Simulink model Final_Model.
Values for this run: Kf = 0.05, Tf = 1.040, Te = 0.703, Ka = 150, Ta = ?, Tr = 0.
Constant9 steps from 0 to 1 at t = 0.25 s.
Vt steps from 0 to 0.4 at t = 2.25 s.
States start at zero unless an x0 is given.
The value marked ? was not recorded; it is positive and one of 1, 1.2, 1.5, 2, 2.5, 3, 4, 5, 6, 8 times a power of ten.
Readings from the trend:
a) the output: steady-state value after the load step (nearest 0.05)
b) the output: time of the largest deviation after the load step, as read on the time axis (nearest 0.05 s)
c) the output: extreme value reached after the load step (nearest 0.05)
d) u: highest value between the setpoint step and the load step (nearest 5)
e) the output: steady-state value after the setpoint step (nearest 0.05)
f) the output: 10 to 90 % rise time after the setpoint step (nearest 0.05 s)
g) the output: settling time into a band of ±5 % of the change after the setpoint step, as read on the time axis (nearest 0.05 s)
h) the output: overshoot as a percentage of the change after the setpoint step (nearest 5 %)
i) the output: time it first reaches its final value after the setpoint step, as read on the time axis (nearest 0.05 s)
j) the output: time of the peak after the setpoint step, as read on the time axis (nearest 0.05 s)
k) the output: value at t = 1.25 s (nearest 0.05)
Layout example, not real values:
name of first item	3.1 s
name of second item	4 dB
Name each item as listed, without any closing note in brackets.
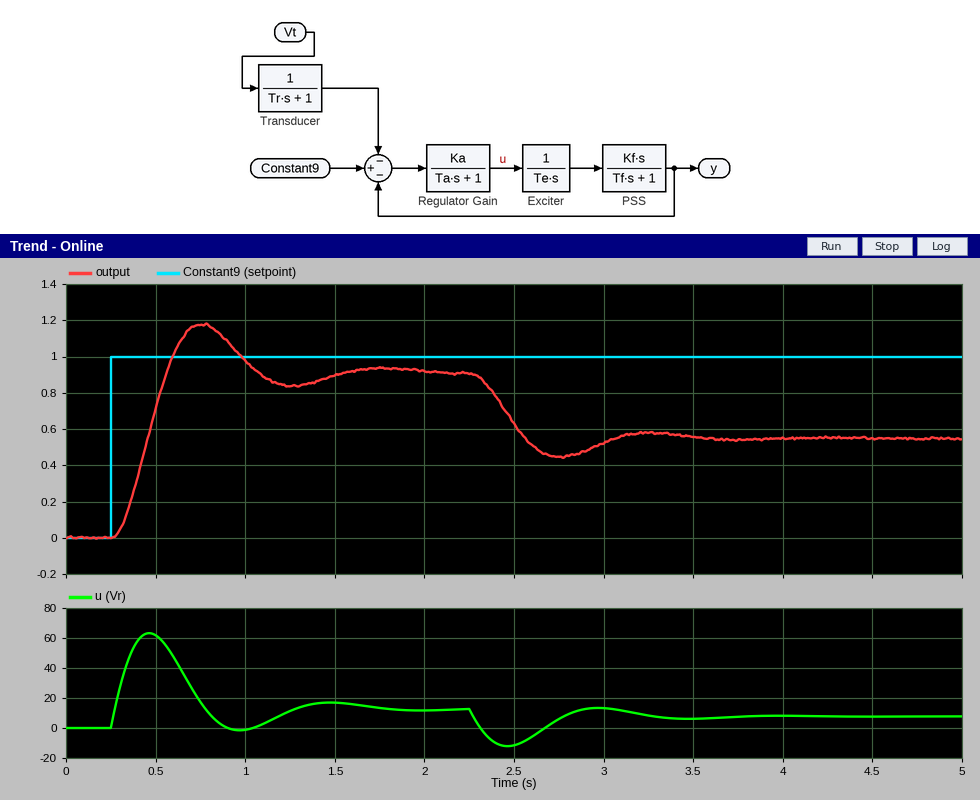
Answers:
the output: steady-state value after the load step	0.55
the output: time of the largest deviation after the load step, as read on the time axis	2.75 s
the output: extreme value reached after the load step	0.45
u: highest value between the setpoint step and the load step	65
the output: steady-state value after the setpoint step	0.90
the output: 10 to 90 % rise time after the setpoint step	0.20 s
the output: settling time into a band of ±5 % of the change after the setpoint step, as read on the time axis	1.40 s
the output: overshoot as a percentage of the change after the setpoint step	30 %
the output: time it first reaches its final value after the setpoint step, as read on the time axis	0.55 s
the output: time of the peak after the setpoint step, as read on the time axis	0.75 s
the output: value at t = 1.25 s	0.85
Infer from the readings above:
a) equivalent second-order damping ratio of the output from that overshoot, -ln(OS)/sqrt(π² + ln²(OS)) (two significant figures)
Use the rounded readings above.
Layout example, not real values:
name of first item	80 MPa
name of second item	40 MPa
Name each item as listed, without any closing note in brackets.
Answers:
equivalent second-order damping ratio of the output from that overshoot, -ln(OS)/sqrt(π² + ln²(OS))	0.36
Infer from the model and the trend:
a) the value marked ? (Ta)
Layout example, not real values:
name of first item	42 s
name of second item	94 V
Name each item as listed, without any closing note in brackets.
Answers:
the value marked ?	0.25
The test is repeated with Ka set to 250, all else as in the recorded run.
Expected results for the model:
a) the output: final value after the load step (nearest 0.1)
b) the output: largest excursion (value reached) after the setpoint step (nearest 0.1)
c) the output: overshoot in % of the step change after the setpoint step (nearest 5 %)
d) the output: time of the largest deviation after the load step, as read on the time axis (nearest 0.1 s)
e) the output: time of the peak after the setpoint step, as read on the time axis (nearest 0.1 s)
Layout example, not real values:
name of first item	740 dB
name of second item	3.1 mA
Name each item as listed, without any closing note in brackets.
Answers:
the output: final value after the load step	0.6
the output: largest excursion (value reached) after the setpoint step	1.3
the output: overshoot in % of the step change after the setpoint step	40 %
the output: time of the largest deviation after the load step, as read on the time axis	2.6 s
the output: time of the peak after the setpoint step, as read on the time axis	0.6 s
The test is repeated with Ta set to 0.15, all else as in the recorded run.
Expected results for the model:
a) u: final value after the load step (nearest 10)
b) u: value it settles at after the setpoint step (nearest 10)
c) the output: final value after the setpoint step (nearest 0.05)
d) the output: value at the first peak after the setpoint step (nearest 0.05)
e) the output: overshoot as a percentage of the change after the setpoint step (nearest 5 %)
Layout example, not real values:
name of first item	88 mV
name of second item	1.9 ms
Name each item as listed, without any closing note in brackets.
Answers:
u: final value after the load step	10
u: value it settles at after the setpoint step	10
the output: final value after the setpoint step	0.90
the output: value at the first peak after the setpoint step	1.10
the output: overshoot as a percentage of the change after the setpoint step	20 %
